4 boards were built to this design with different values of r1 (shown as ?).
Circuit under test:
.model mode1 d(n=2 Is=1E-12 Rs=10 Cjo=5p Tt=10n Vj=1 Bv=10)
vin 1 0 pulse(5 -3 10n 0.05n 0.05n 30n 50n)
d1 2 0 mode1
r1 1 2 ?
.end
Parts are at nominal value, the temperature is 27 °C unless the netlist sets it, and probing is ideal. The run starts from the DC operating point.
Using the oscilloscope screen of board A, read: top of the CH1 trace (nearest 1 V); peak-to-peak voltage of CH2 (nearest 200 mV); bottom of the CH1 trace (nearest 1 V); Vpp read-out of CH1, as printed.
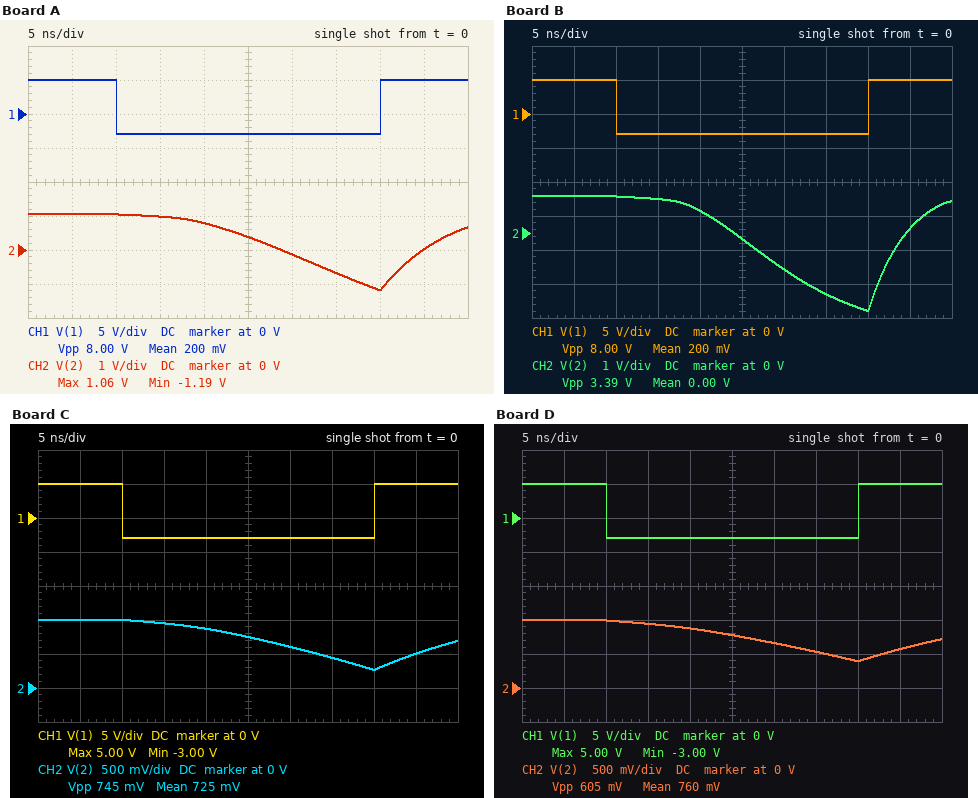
5 V
2.2 V
-3 V
8.00 V
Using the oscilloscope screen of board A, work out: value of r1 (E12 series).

5.6 kΩ
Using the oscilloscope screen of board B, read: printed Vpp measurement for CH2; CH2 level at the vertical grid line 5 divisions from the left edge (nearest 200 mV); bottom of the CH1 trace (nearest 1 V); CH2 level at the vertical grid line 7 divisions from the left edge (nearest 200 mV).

3.39 V
-200 mV
-3 V
-1.8 V
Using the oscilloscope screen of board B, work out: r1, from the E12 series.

3.3 kΩ
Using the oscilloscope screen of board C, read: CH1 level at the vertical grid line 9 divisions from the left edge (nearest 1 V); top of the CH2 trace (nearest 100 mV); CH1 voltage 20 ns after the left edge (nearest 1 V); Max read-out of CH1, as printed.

5 V
1.0 V
-3 V
5.00 V
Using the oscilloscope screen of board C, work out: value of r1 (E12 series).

15 kΩ
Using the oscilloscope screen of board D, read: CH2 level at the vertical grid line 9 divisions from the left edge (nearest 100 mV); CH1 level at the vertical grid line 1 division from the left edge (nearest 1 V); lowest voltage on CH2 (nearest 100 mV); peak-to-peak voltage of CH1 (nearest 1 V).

600 mV
5 V
400 mV
8 V
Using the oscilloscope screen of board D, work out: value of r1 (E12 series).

18 kΩ
